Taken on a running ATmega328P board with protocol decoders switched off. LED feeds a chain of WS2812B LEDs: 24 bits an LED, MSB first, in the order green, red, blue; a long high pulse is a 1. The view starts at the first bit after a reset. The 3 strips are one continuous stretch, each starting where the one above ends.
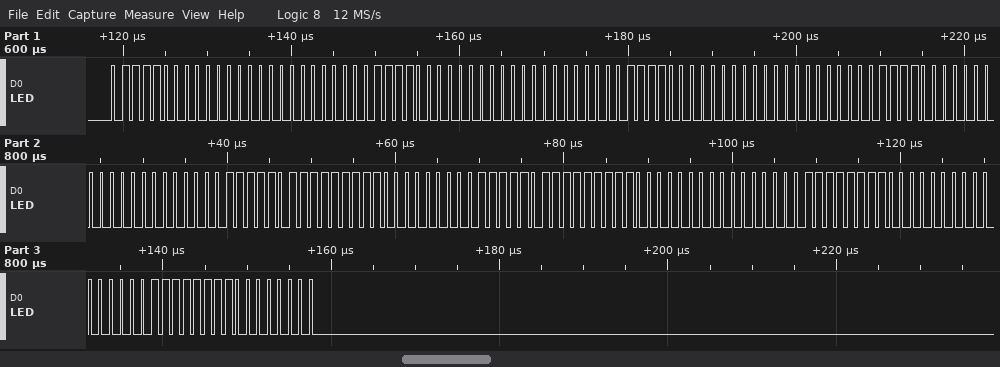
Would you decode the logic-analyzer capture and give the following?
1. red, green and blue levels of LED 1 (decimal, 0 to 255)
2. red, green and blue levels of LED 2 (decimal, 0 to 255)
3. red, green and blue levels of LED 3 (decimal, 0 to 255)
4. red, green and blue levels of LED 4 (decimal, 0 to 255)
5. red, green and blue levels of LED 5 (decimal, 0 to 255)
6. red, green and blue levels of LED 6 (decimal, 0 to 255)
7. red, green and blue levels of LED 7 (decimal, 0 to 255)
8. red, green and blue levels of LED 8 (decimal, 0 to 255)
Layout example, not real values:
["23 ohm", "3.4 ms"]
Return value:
["0, 120, 0", "0, 120, 0", "0, 120, 0", "0, 120, 0", "255, 125, 0", "255, 125, 0", "255, 0, 0", "255, 0, 0"]
